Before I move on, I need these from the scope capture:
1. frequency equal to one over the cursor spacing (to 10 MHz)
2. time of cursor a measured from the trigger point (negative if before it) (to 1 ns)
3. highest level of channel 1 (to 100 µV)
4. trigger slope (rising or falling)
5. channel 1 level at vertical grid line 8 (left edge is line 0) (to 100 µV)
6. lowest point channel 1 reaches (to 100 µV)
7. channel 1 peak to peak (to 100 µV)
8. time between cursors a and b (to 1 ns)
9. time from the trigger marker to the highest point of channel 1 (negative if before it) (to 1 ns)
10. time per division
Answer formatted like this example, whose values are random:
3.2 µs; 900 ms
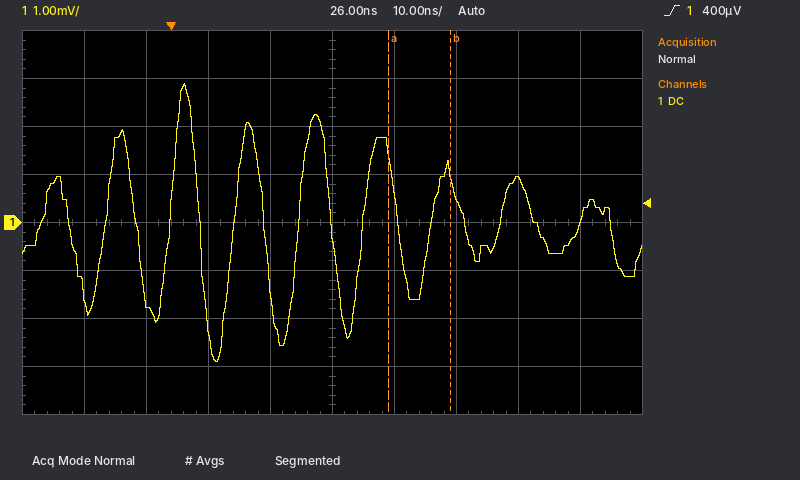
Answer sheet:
100 MHz; +35 ns; 2.9 mV; rising; 900 µV; -2.9 mV; 5.8 mV; 10 ns; +2 ns; 10 ns
